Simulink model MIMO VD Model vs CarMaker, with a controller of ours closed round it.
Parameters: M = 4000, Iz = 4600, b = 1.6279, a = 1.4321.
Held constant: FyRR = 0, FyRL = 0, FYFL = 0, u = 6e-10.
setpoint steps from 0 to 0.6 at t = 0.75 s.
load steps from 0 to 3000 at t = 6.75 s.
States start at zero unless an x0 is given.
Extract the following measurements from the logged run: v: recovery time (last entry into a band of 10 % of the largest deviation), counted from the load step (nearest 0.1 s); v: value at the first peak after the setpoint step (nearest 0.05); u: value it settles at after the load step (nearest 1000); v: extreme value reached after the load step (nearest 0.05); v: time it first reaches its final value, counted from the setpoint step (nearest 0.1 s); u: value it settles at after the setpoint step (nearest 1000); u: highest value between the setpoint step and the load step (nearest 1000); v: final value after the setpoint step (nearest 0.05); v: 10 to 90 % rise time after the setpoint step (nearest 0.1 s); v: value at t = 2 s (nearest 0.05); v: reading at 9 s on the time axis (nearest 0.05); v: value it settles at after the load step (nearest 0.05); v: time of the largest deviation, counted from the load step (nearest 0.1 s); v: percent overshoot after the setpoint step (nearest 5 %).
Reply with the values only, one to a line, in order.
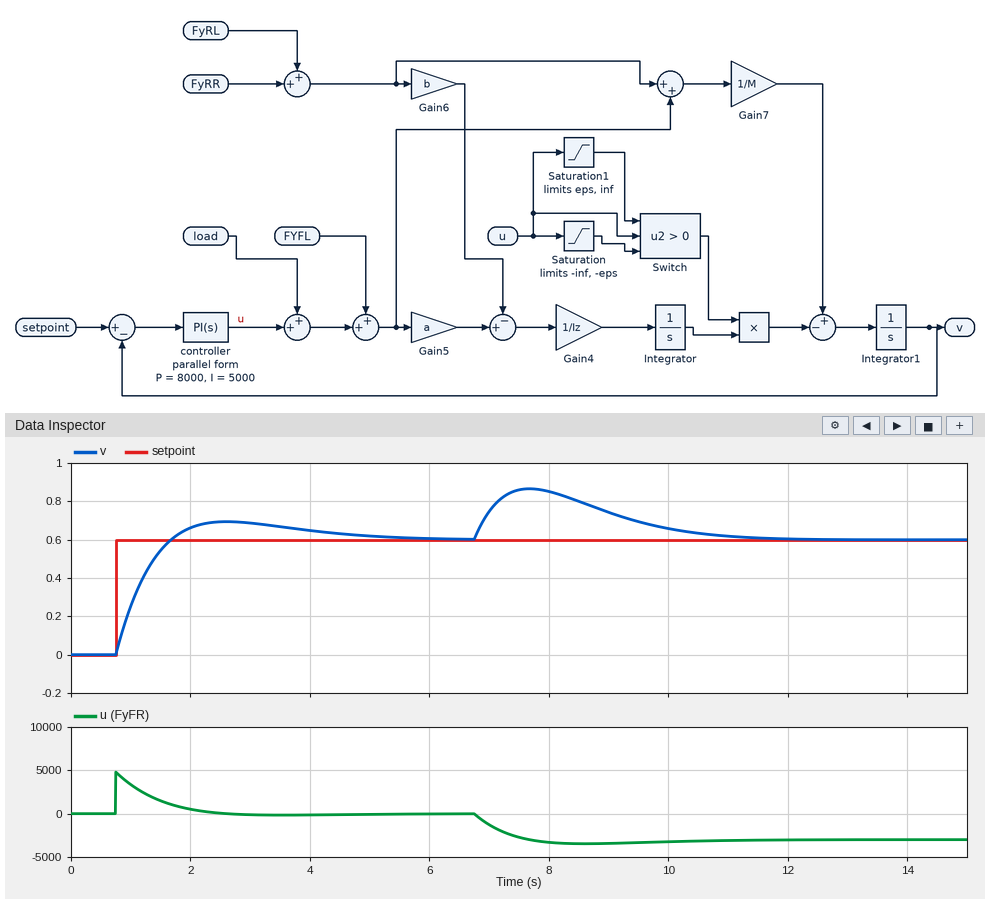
4.0 s
0.70
-3000
0.85
0.9 s
0
5000
0.60
0.7 s
0.65
0.75
0.60
0.9 s
15 %
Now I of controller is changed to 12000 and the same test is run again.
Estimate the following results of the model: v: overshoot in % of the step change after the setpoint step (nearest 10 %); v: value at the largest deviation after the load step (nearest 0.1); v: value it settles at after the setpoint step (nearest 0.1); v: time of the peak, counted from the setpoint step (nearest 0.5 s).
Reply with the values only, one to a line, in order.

30 %
0.8
0.6
1.5 s
